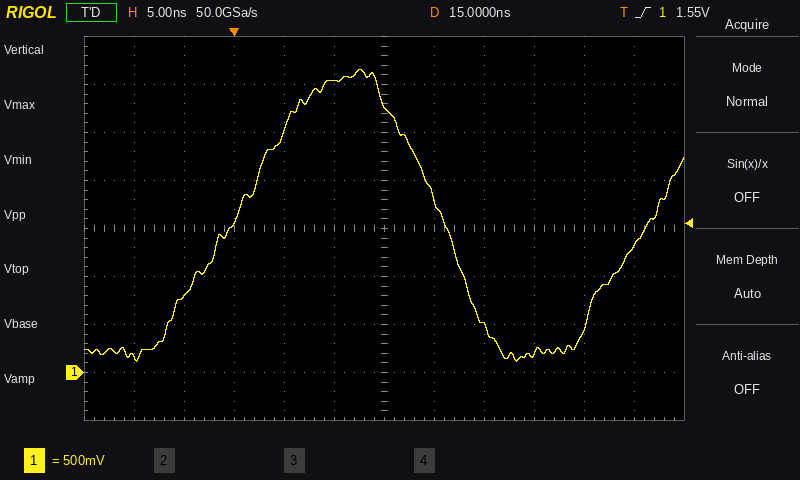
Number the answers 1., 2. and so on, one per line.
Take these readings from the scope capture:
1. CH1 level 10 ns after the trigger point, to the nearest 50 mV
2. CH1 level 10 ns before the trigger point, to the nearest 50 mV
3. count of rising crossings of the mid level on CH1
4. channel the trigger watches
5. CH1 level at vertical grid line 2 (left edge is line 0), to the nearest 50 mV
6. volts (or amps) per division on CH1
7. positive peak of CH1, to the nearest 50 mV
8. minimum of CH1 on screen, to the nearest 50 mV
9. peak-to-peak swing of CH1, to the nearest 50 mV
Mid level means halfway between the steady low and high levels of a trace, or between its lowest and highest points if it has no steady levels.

1. 3.05 V
2. 150 mV
3. 2
4. CH1
5. 800 mV
6. 500 mV
7. 3.15 V
8. 100 mV
9. 3.05 V
